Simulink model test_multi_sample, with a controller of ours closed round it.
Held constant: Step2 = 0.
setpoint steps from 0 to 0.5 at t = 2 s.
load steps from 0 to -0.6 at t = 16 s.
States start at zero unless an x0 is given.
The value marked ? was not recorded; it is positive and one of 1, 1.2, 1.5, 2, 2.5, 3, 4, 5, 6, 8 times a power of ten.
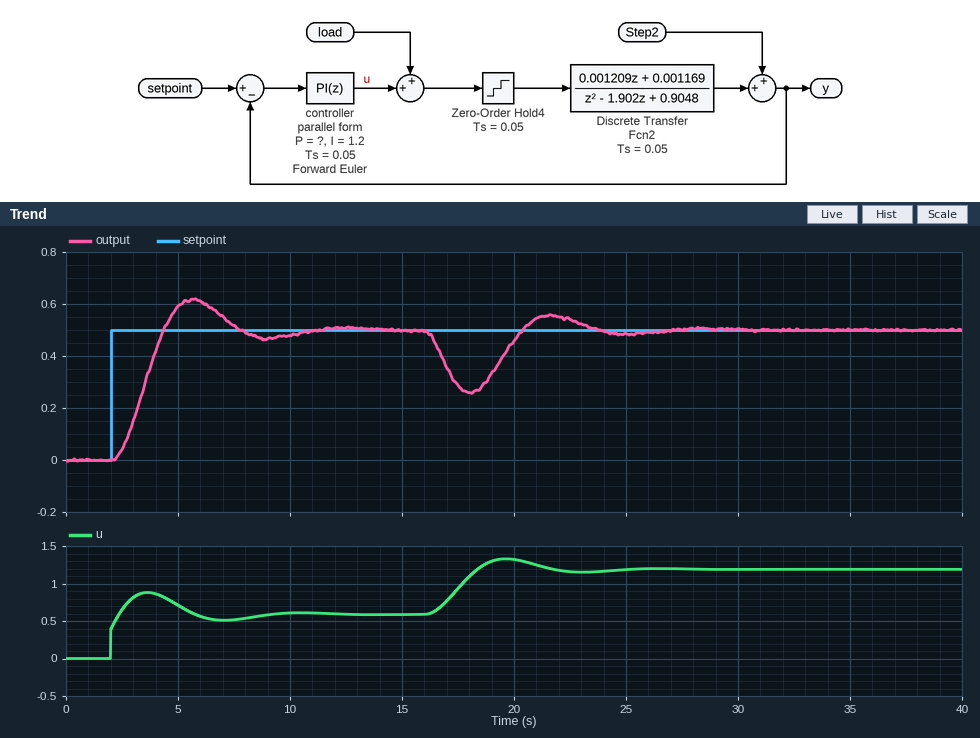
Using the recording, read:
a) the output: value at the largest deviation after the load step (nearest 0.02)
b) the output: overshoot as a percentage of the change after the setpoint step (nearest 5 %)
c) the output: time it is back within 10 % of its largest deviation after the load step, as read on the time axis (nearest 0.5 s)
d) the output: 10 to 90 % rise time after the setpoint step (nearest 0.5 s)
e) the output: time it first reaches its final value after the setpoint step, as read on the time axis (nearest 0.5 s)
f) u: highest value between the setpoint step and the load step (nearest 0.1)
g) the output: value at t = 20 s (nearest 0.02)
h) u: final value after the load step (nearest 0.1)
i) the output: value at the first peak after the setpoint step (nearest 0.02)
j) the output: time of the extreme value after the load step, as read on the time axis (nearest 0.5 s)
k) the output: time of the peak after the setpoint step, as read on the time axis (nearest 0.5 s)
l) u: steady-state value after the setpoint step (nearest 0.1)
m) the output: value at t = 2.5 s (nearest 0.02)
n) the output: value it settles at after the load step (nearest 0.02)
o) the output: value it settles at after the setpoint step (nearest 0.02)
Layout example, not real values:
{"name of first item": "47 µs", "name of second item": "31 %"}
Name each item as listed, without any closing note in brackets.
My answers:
{"the output: value at the largest deviation after the load step": "0.26", "the output: overshoot as a percentage of the change after the setpoint step": "25 %", "the output: time it is back within 10 % of its largest deviation after the load step, as read on the time axis": "23.0 s", "the output: 10 to 90 % rise time after the setpoint step": "1.5 s", "the output: time it first reaches its final value after the setpoint step, as read on the time axis": "4.5 s", "u: highest value between the setpoint step and the load step": "0.9", "the output: value at t = 20 s": "0.46", "u: final value after the load step": "1.2", "the output: value at the first peak after the setpoint step": "0.62", "the output: time of the extreme value after the load step, as read on the time axis": "18.0 s", "the output: time of the peak after the setpoint step, as read on the time axis": "5.5 s", "u: steady-state value after the setpoint step": "0.6", "the output: value at t = 2.5 s": "0.04", "the output: value it settles at after the load step": "0.50", "the output: value it settles at after the setpoint step": "0.50"}
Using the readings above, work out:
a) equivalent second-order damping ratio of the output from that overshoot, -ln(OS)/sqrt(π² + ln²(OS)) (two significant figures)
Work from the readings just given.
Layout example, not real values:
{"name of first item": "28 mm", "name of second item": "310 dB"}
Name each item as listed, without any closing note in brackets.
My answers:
{"equivalent second-order damping ratio of the output from that overshoot, -ln(OS)/sqrt(π² + ln²(OS))": "0.40"}
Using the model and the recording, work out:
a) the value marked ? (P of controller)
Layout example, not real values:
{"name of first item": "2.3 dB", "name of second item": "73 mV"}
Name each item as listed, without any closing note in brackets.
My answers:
{"the value marked ?": "0.8"}
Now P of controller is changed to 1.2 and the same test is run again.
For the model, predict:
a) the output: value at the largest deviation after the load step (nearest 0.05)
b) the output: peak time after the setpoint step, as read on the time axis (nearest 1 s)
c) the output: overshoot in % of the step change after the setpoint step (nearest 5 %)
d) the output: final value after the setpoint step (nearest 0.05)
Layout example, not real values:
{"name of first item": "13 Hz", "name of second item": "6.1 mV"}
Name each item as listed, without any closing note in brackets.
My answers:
{"the output: value at the largest deviation after the load step": "0.30", "the output: peak time after the setpoint step, as read on the time axis": "5 s", "the output: overshoot in % of the step change after the setpoint step": "15 %", "the output: final value after the setpoint step": "0.50"}
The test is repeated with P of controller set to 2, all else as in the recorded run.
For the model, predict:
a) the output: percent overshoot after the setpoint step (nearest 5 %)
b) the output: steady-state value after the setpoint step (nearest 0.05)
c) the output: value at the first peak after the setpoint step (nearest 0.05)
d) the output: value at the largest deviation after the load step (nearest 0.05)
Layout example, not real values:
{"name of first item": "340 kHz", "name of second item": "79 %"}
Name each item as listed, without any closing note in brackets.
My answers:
{"the output: percent overshoot after the setpoint step": "10 %", "the output: steady-state value after the setpoint step": "0.50", "the output: value at the first peak after the setpoint step": "0.55", "the output: value at the largest deviation after the load step": "0.30"}
